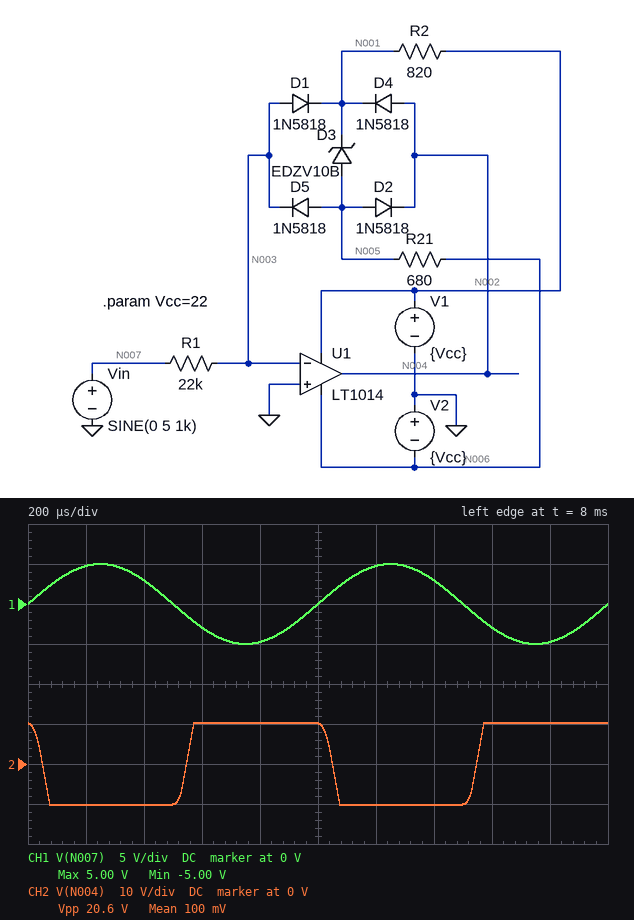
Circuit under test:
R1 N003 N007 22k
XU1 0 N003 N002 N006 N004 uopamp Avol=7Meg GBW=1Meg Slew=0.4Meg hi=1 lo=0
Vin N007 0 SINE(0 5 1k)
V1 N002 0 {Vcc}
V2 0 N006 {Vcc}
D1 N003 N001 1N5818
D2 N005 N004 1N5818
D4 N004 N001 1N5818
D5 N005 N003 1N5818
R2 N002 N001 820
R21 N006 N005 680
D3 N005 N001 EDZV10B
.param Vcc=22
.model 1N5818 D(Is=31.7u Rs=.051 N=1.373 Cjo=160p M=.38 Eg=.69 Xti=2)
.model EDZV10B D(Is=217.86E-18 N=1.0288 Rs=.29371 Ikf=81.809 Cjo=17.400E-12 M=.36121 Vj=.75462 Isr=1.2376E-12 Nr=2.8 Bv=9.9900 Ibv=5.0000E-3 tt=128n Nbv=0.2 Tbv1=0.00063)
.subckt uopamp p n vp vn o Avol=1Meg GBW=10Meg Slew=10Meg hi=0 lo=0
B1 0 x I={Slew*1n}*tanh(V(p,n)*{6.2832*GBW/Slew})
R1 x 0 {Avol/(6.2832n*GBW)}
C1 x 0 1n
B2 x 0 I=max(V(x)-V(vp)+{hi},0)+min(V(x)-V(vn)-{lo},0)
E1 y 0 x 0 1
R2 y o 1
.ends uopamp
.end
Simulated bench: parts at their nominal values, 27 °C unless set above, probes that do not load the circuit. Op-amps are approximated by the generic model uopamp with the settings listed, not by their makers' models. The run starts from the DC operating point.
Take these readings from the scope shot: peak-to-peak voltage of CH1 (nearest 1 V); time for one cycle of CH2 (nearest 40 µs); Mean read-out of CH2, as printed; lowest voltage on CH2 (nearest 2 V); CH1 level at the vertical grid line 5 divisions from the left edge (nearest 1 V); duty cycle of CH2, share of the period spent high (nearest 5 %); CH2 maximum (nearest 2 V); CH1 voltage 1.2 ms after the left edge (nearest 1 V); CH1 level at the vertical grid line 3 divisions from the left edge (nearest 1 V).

10 V
1.00 ms
100 mV
-10 V
0 V
50 %
10 V
5 V
-3 V
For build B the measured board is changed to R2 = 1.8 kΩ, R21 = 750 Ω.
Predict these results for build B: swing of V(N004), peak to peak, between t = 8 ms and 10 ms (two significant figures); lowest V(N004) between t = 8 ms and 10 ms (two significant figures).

10 V
96 mV
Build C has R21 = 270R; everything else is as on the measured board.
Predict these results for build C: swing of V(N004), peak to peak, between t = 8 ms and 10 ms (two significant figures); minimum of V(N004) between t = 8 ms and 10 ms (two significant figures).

10 V
150 mV
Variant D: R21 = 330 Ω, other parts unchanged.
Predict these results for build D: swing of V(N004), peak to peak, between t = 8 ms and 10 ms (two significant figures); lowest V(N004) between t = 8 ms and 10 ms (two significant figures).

10 V
130 mV
